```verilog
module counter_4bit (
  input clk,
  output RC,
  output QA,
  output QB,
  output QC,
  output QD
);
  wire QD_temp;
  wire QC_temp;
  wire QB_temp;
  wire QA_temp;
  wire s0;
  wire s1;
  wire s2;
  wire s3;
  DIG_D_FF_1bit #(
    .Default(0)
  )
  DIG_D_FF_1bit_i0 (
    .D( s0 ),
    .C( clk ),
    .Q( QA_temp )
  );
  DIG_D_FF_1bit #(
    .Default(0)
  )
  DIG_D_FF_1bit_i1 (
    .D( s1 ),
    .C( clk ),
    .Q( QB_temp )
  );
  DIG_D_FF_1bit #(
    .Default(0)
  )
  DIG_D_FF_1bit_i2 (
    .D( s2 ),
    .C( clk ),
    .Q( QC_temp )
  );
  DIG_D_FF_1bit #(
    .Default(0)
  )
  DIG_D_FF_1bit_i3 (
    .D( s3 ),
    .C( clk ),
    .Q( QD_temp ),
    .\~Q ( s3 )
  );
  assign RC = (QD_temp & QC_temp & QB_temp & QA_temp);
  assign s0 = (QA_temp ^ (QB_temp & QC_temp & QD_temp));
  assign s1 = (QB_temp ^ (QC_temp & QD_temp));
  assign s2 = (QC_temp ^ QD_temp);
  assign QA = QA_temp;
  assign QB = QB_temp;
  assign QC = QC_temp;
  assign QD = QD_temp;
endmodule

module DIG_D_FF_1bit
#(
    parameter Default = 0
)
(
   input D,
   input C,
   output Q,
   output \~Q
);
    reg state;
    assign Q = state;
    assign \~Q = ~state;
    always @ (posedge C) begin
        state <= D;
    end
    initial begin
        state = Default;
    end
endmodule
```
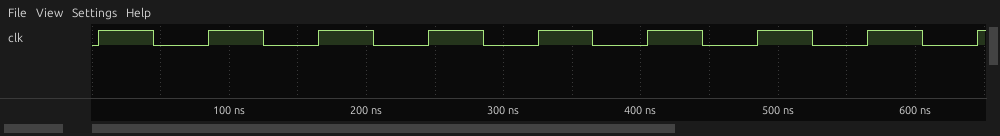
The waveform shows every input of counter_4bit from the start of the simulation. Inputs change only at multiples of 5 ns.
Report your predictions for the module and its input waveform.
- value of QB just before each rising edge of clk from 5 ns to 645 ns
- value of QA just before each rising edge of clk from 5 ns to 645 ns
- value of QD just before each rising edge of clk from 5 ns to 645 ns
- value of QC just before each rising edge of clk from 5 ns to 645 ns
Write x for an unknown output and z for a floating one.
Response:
0 0 0 0 1 1 1 1 0
0 0 0 0 0 0 0 0 1
0 1 0 1 0 1 0 1 0
0 0 1 1 0 0 1 1 0
